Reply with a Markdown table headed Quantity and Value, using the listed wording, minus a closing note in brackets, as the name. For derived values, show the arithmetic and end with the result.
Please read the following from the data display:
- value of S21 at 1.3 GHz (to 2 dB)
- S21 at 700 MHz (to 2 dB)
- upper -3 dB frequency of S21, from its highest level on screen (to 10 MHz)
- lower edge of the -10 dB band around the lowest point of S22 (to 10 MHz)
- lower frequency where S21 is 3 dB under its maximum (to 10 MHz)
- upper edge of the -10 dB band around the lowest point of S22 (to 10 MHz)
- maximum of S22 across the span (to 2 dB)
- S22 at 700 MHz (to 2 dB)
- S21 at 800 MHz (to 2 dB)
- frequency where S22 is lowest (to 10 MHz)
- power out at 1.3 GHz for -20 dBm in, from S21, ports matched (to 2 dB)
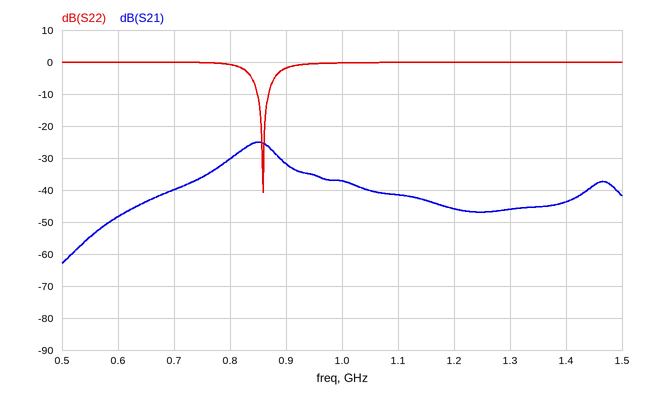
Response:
| Quantity | Value |
|---|---|
| value of S21 at 1.3 GHz | -46 dB |
| S21 at 700 MHz | -40 dB |
| upper -3 dB frequency of S21, from its highest level on screen | 880 MHz |
| lower edge of the -10 dB band around the lowest point of S22 | 850 MHz |
| lower frequency where S21 is 3 dB under its maximum | 820 MHz |
| upper edge of the -10 dB band around the lowest point of S22 | 870 MHz |
| maximum of S22 across the span | 0 dB |
| S22 at 700 MHz | 0 dB |
| S21 at 800 MHz | -30 dB |
| frequency where S22 is lowest | 860 MHz |
| power out at 1.3 GHz for -20 dBm in, from S21, ports matched | -20 dBm + (-46 dB) = -66 dBm |
